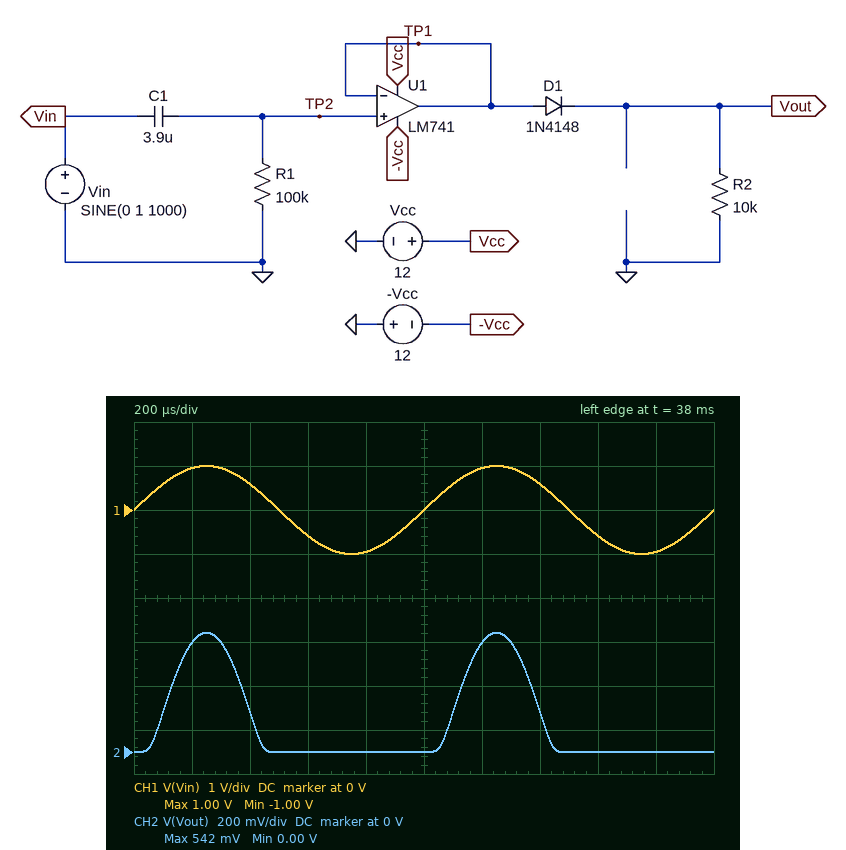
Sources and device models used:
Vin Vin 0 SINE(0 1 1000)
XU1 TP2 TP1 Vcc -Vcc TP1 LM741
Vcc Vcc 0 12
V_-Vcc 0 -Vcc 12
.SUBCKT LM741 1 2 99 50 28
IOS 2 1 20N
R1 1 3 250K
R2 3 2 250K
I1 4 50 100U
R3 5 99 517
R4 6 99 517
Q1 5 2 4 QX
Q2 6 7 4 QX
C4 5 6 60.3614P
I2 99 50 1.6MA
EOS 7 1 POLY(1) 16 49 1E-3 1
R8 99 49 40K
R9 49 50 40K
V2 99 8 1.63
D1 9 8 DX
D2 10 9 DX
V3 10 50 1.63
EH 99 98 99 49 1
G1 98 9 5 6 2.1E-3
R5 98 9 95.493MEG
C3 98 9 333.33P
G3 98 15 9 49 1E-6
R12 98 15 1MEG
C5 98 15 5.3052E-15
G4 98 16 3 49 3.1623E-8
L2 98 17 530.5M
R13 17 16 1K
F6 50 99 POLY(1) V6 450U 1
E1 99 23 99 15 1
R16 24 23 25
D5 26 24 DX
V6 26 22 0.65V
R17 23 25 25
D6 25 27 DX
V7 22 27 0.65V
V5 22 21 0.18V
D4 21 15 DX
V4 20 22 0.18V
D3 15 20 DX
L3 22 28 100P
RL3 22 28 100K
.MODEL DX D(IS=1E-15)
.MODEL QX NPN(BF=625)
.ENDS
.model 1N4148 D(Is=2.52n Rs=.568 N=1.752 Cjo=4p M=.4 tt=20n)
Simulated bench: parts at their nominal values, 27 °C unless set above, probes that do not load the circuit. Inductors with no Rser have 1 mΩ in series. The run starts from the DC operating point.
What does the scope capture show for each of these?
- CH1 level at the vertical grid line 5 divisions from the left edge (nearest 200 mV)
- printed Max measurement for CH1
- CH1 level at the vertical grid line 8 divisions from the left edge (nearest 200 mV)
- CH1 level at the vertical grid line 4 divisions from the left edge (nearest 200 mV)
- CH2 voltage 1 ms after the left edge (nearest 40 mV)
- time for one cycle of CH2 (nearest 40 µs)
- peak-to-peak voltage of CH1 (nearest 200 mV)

0 V
1.00 V
-600 mV
-1.0 V
0 V
1.00 ms
2.0 V
